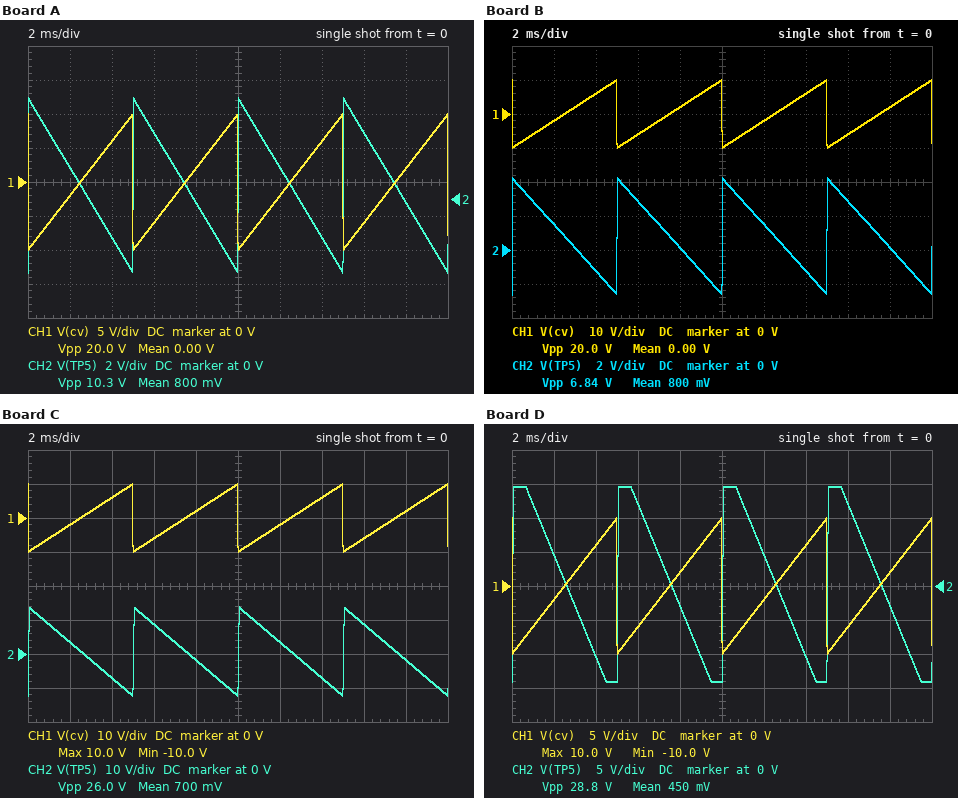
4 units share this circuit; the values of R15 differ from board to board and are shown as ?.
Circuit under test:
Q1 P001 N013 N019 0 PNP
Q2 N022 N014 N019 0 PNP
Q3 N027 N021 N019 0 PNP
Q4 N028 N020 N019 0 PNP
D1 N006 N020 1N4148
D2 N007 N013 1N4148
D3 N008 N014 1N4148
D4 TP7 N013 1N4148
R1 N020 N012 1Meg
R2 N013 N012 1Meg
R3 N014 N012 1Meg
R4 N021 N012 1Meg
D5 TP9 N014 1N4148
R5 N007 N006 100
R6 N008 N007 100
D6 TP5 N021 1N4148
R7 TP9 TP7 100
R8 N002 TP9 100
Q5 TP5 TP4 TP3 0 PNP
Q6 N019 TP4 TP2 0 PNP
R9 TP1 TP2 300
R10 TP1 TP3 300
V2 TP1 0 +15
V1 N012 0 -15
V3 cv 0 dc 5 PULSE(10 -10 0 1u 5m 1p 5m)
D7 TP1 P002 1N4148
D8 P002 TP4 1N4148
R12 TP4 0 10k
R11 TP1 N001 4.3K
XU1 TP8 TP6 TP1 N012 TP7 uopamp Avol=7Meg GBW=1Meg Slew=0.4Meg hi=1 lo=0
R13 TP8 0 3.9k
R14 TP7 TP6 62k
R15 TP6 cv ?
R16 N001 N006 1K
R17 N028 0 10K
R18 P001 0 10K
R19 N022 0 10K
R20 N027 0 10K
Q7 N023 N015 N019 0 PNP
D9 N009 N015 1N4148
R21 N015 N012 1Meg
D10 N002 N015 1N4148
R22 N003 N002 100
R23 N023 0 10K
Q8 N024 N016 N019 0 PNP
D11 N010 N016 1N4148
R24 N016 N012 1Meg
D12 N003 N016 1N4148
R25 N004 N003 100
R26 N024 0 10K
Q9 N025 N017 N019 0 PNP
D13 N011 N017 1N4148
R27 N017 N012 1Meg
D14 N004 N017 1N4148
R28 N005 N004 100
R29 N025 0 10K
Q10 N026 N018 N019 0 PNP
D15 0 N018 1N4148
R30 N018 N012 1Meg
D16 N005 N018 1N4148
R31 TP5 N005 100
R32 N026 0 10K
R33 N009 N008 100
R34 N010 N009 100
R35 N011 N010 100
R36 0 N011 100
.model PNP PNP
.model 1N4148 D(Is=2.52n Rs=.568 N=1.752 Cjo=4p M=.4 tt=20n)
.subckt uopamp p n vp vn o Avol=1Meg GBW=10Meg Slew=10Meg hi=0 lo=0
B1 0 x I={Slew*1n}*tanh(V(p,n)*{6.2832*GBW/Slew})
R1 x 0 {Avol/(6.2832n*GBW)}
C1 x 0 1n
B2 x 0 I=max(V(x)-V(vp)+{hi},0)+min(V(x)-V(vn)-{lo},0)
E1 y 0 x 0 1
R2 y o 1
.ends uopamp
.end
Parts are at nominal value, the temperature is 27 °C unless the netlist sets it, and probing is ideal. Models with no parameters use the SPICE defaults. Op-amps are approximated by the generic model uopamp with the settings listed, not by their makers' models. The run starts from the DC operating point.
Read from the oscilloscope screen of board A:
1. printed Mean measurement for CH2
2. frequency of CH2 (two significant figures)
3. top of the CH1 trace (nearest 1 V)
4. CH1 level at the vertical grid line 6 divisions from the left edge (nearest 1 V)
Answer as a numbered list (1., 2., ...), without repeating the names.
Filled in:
1. 800 mV
2. 200 Hz
3. 10 V
4. -2 V
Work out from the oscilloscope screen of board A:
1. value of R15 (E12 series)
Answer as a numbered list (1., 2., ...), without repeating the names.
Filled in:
1. 120 kΩ
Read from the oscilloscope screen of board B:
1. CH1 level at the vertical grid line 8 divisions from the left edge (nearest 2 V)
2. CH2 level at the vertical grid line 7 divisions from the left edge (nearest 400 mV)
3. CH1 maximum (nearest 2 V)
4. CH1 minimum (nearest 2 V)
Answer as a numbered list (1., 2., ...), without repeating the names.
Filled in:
1. -6 V
2. -1.2 V
3. 10 V
4. -10 V
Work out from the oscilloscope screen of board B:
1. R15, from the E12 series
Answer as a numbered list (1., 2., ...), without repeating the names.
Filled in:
1. 180 kΩ
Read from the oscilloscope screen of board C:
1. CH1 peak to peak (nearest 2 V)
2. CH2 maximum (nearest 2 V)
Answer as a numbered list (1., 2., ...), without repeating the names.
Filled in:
1. 20 V
2. 14 V
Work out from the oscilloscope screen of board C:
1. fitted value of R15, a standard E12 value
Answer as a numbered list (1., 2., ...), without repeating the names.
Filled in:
1. 47 kΩ
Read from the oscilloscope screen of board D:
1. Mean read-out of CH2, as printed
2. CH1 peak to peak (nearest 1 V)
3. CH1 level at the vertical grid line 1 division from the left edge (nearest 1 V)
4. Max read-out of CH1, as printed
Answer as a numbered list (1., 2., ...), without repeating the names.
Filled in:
1. 450 mV
2. 20 V
3. -2 V
4. 10.0 V
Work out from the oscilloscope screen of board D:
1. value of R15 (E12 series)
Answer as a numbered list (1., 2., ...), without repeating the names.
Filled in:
1. 33 kΩ
